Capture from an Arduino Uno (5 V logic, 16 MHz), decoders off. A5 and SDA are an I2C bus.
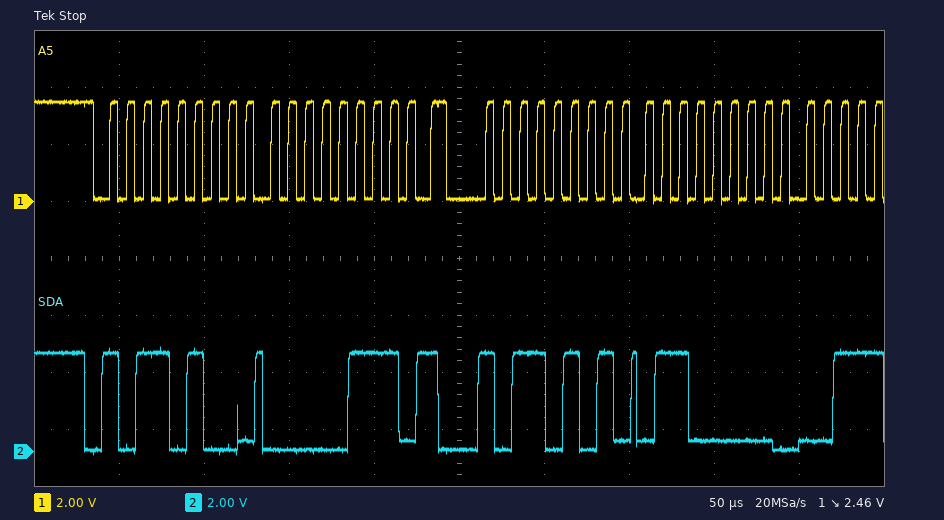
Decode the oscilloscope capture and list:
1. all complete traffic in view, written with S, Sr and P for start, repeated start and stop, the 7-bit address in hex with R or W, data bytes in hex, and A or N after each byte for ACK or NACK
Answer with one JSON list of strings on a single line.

["S 5AW A 07 A Sr 5AR A 60 A"]
